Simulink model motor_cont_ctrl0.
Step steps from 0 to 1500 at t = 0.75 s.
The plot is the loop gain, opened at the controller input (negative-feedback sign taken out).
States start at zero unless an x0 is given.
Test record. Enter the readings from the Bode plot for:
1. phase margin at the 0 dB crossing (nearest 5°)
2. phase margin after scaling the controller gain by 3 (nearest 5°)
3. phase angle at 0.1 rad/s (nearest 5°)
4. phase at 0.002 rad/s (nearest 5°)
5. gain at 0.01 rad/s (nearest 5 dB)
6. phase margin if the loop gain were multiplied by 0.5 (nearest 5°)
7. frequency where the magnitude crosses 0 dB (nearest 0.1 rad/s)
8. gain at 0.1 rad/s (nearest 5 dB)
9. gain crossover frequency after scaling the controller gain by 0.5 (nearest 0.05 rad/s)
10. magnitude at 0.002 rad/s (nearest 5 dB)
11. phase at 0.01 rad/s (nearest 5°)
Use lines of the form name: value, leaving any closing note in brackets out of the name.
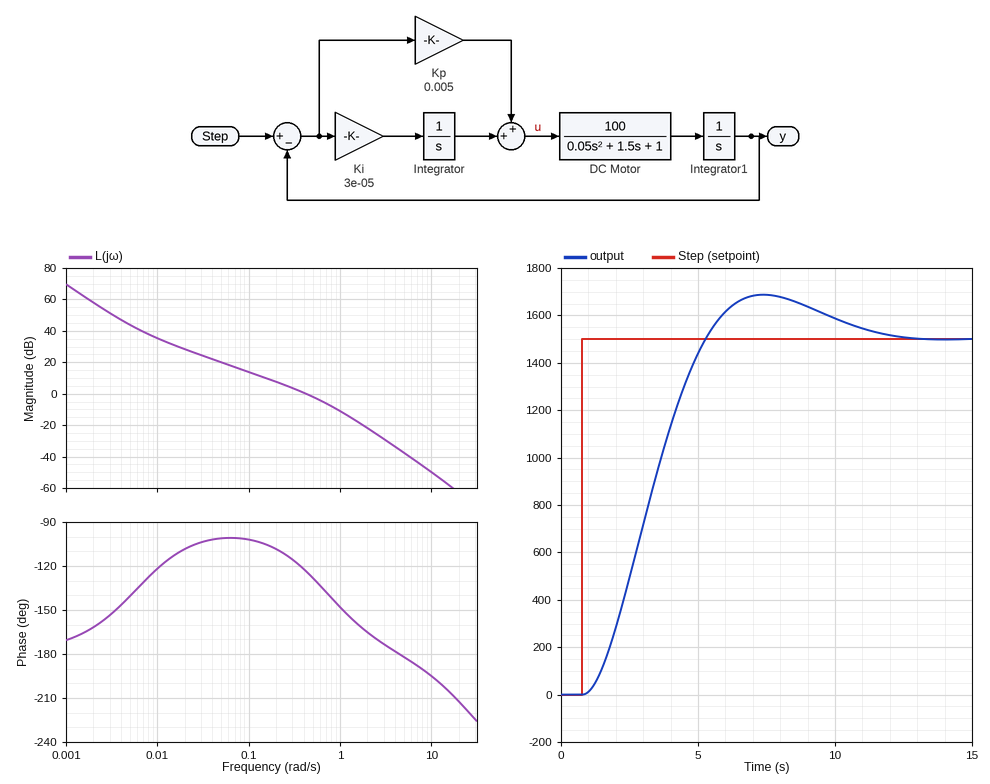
phase margin at the 0 dB crossing: 55°
phase margin after scaling the controller gain by 3: 35°
phase angle at 0.1 rad/s: -100°
phase at 0.002 rad/s: -160°
gain at 0.01 rad/s: 35 dB
phase margin if the loop gain were multiplied by 0.5: 70°
frequency where the magnitude crosses 0 dB: 0.4 rad/s
gain at 0.1 rad/s: 15 dB
gain crossover frequency after scaling the controller gain by 0.5: 0.25 rad/s
magnitude at 0.002 rad/s: 60 dB
phase at 0.01 rad/s: -120°
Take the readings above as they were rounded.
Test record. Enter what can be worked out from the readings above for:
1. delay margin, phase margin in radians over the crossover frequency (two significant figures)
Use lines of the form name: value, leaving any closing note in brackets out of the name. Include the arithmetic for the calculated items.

delay margin, phase margin in radians over the crossover frequency: 55 × π / 180 / 0.4 = 2.4 s
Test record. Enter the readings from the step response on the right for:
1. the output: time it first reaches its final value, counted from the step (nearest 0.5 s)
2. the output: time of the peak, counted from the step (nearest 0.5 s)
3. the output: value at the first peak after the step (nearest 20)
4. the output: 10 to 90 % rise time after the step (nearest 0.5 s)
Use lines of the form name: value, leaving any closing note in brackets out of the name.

the output: time it first reaches its final value, counted from the step: 4.5 s
the output: time of the peak, counted from the step: 6.5 s
the output: value at the first peak after the step: 1680
the output: 10 to 90 % rise time after the step: 3.0 s
